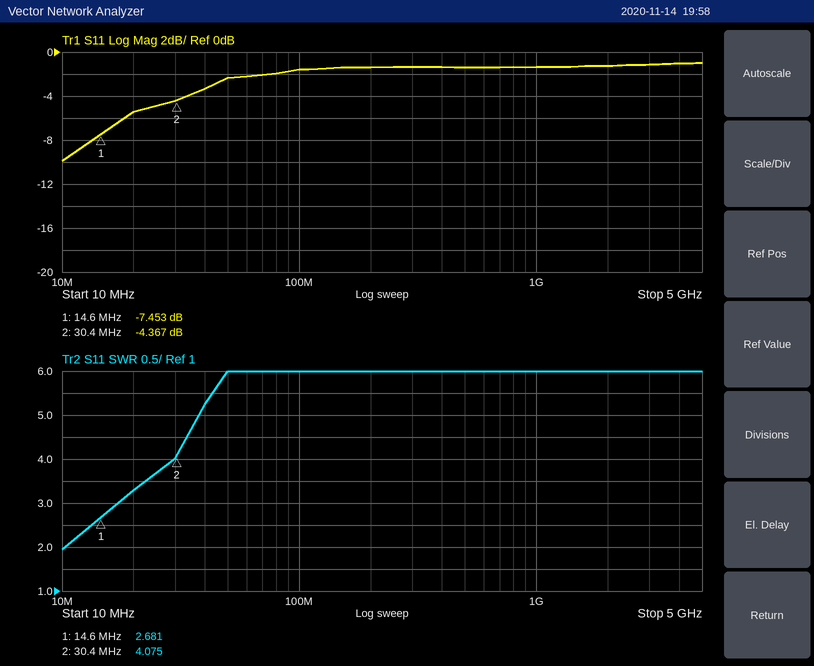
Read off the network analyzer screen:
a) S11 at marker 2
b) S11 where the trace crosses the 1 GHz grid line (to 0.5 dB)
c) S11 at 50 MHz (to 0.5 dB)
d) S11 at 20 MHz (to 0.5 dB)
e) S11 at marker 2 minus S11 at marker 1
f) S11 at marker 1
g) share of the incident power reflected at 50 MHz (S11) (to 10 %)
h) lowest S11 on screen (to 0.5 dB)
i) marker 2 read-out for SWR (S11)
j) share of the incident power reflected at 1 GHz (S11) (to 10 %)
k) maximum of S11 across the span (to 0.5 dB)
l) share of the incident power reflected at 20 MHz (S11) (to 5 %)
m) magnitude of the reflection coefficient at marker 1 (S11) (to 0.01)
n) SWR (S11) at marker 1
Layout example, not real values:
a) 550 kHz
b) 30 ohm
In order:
a) -4.367 dB
b) -1.5 dB
c) -2.5 dB
d) -5.5 dB
e) 3.086 dB
f) -7.453 dB
g) 60 %
h) -10.0 dB
i) 4.075
j) 70 %
k) -1.0 dB
l) 30 %
m) 0.42
n) 2.681
